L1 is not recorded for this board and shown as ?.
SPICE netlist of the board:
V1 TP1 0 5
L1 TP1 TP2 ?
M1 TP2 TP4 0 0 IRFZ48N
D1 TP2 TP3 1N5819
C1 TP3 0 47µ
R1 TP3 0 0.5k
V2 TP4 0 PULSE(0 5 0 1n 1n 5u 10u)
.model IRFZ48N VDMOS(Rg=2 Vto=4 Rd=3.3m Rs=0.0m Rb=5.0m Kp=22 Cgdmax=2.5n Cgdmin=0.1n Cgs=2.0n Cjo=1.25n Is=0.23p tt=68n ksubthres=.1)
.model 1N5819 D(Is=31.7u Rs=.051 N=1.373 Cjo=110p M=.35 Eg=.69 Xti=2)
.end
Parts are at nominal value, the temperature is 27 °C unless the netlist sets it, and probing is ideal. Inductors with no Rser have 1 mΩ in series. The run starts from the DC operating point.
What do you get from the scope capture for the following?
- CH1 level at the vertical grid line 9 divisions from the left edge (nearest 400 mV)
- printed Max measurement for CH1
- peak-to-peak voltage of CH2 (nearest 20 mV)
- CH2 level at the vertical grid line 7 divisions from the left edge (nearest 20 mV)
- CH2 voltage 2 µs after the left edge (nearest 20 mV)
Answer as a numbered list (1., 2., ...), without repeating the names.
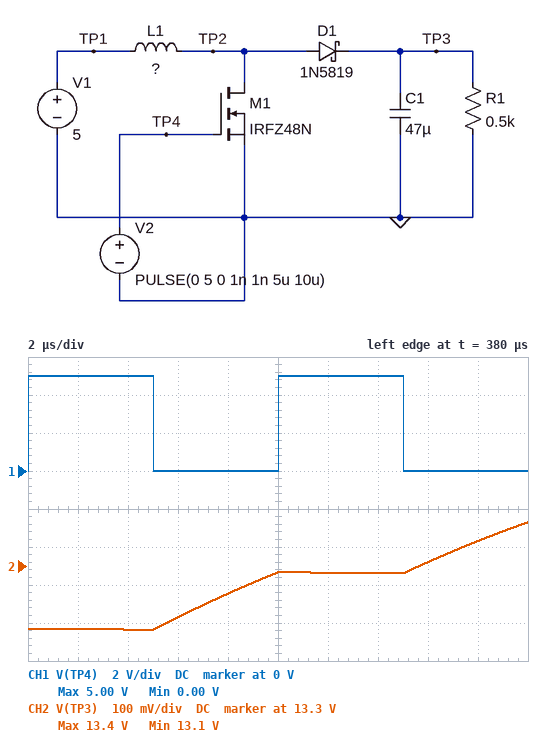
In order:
1. 0 V
2. 5.00 V
3. 280 mV
4. 13.28 V
5. 13.14 V
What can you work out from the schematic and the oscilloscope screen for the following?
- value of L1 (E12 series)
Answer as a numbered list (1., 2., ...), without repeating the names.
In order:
1. 120 µH
